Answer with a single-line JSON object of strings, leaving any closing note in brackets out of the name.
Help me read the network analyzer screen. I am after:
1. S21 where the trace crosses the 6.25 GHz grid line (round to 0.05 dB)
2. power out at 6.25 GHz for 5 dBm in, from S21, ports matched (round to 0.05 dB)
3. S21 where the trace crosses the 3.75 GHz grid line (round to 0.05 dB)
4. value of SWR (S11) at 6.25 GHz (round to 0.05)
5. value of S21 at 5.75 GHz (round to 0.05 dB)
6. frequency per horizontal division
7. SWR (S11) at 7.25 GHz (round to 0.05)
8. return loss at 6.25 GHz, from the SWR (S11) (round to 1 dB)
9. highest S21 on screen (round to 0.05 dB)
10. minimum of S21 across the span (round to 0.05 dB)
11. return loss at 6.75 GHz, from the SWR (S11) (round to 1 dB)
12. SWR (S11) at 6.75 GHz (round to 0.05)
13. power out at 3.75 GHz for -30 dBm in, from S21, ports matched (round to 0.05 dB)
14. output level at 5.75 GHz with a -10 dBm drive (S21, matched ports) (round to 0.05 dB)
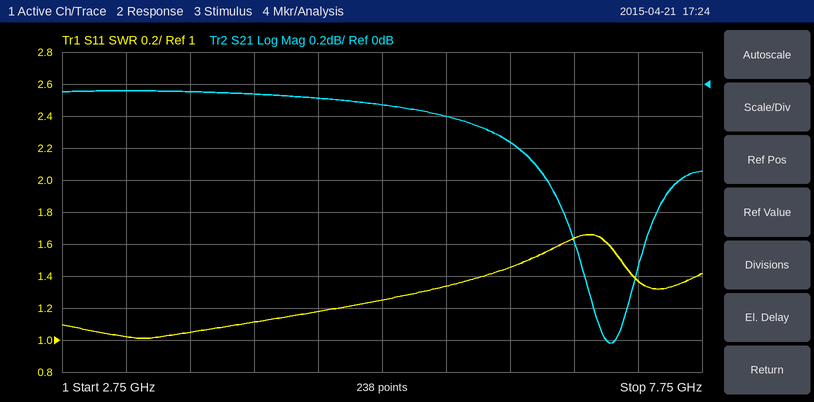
{"S21 where the trace crosses the 6.25 GHz grid line": "-0.35 dB", "power out at 6.25 GHz for 5 dBm in, from S21, ports matched": "4.65 dBm", "S21 where the trace crosses the 3.75 GHz grid line": "-0.05 dB", "value of SWR (S11) at 6.25 GHz": "1.45", "value of S21 at 5.75 GHz": "-0.20 dB", "frequency per horizontal division": "500 MHz", "SWR (S11) at 7.25 GHz": "1.35", "return loss at 6.25 GHz, from the SWR (S11)": "15 dB", "highest S21 on screen": "-0.05 dB", "minimum of S21 across the span": "-1.60 dB", "return loss at 6.75 GHz, from the SWR (S11)": "12 dB", "SWR (S11) at 6.75 GHz": "1.65", "power out at 3.75 GHz for -30 dBm in, from S21, ports matched": "-30.05 dBm", "output level at 5.75 GHz with a -10 dBm drive (S21, matched ports)": "-10.20 dBm"}
